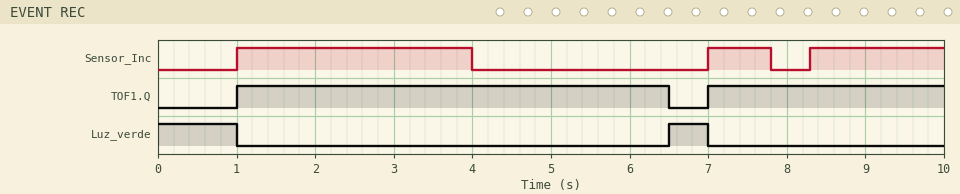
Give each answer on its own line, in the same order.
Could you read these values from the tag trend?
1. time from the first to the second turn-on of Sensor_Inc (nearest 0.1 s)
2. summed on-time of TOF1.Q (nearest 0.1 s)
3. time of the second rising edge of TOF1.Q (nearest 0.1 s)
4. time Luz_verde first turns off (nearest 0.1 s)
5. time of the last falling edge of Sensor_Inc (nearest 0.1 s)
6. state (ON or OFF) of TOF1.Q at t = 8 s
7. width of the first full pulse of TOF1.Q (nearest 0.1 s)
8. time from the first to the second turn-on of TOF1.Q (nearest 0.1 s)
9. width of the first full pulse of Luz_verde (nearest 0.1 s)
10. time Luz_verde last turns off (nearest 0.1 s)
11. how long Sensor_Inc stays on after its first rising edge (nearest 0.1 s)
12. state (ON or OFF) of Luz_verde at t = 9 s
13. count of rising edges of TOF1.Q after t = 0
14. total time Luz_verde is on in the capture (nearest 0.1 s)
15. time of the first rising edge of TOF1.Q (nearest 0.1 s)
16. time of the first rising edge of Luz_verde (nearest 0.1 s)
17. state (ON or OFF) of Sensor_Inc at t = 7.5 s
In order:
6.0 s
8.5 s
7.0 s
1.0 s
7.8 s
ON
5.5 s
6.0 s
0.5 s
7.0 s
3.0 s
OFF
2
1.5 s
1.0 s
6.5 s
ON
